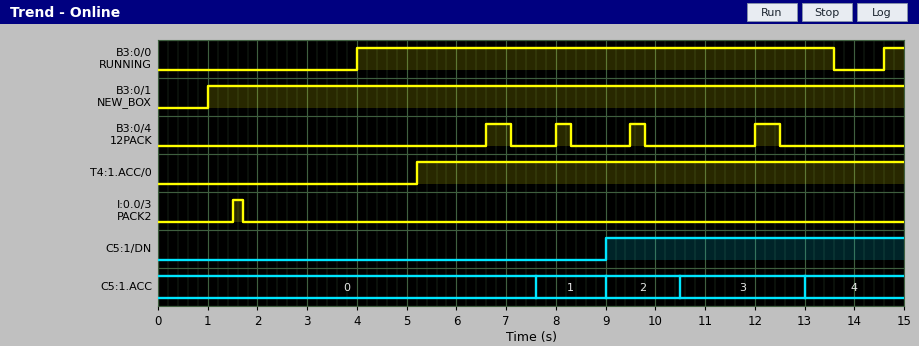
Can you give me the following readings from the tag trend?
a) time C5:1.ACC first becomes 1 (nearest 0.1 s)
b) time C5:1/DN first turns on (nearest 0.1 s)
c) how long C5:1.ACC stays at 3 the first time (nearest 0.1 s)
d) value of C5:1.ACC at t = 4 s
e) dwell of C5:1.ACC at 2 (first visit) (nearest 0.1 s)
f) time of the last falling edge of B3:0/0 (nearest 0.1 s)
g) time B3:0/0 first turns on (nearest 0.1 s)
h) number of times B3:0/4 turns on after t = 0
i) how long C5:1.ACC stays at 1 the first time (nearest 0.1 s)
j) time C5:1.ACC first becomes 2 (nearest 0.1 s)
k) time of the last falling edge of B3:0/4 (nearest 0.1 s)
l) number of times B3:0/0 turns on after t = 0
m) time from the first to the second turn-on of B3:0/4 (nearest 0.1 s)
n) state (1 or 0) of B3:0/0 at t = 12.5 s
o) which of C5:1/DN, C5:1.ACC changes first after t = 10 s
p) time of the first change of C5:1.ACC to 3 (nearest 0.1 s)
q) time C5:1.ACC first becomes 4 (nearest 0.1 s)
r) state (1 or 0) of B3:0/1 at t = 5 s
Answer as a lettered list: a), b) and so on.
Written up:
a) 7.6 s
b) 9.0 s
c) 2.5 s
d) 0
e) 1.5 s
f) 13.6 s
g) 4.0 s
h) 4
i) 1.4 s
j) 9.0 s
k) 12.5 s
l) 2
m) 1.4 s
n) 1
o) C5:1.ACC
p) 10.5 s
q) 13.0 s
r) 1
